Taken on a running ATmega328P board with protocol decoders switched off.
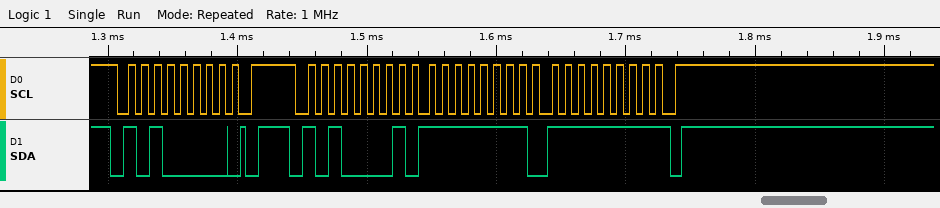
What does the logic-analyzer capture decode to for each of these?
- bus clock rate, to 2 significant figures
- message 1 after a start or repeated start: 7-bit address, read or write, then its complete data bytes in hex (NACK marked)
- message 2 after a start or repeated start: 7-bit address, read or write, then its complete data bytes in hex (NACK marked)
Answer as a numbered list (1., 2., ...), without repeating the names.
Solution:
1. 100 kHz
2. 0x50 write
3. 0x50 read: FF FF NACK
